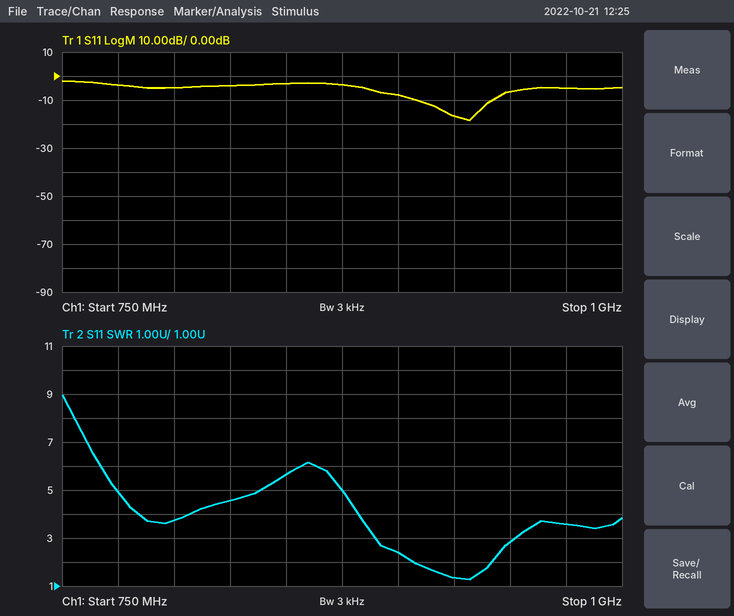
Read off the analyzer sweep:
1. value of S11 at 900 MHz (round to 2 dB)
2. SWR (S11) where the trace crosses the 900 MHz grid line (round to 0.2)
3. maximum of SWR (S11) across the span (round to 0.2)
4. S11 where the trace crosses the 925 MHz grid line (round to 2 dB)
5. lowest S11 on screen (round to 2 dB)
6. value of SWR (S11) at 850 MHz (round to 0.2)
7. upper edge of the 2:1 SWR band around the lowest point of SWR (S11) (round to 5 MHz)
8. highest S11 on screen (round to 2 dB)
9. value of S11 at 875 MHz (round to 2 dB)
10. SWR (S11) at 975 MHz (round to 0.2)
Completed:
-8 dB
2.4
9.0
-16 dB
-18 dB
5.6
940 MHz
-2 dB
-4 dB
3.6
